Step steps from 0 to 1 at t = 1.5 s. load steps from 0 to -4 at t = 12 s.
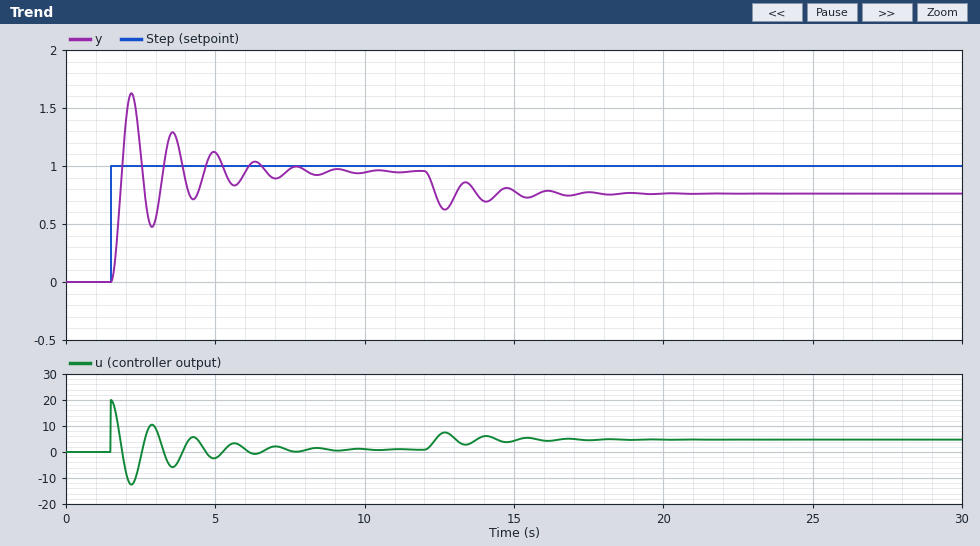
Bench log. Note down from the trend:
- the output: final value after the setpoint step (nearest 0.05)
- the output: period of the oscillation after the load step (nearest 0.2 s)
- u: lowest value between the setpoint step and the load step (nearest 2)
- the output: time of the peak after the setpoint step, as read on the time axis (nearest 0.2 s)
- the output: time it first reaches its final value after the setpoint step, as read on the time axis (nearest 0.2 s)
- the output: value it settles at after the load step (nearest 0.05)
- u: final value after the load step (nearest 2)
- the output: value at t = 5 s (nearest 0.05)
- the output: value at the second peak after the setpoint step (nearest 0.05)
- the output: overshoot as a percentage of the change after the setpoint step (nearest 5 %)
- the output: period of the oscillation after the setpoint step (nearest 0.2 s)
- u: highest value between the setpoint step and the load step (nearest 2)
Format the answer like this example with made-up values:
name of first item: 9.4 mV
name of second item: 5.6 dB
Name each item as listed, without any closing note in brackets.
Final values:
the output: final value after the setpoint step: 0.95
the output: period of the oscillation after the load step: 1.4 s
u: lowest value between the setpoint step and the load step: -12
the output: time of the peak after the setpoint step, as read on the time axis: 2.2 s
the output: time it first reaches its final value after the setpoint step, as read on the time axis: 1.8 s
the output: value it settles at after the load step: 0.75
u: final value after the load step: 4
the output: value at t = 5 s: 1.10
the output: value at the second peak after the setpoint step: 1.30
the output: overshoot as a percentage of the change after the setpoint step: 70 %
the output: period of the oscillation after the setpoint step: 1.4 s
u: highest value between the setpoint step and the load step: 20
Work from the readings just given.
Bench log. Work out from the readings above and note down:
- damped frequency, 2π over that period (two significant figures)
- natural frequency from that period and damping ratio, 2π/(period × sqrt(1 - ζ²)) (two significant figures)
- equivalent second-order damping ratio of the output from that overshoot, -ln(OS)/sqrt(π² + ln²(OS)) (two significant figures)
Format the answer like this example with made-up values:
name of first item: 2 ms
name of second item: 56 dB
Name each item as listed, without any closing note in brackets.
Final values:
damped frequency, 2π over that period: 4.5 rad/s
natural frequency from that period and damping ratio, 2π/(period × sqrt(1 - ζ²)): 4.5 rad/s
equivalent second-order damping ratio of the output from that overshoot, -ln(OS)/sqrt(π² + ln²(OS)): 0.11
